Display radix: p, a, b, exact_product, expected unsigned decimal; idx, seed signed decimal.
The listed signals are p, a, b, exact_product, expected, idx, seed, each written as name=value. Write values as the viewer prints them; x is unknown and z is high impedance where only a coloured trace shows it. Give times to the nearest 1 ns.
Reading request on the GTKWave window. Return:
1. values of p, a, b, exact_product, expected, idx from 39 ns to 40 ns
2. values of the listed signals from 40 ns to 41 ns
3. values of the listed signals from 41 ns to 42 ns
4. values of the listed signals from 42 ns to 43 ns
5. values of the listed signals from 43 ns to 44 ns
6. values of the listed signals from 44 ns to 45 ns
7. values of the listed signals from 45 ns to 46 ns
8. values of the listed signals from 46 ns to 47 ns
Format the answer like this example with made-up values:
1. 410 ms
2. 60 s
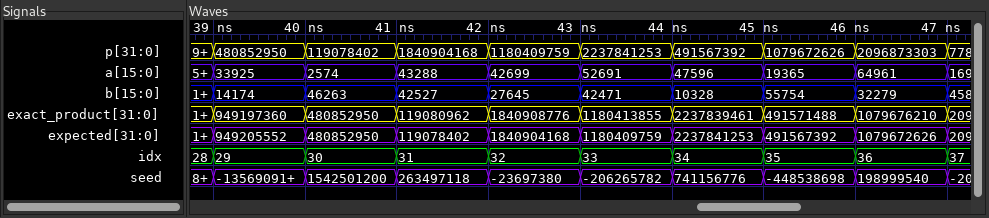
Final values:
1. p=480852950, a=33925, b=14174, exact_product=949197360, expected=949205552, idx=29
2. p=119078402, a=2574, b=46263, exact_product=480852950, expected=480852950, idx=30, seed=1542501200
3. p=1840904168, a=43288, b=42527, exact_product=119080962, expected=119078402, idx=31, seed=263497118
4. p=1180409759, a=42699, b=27645, exact_product=1840908776, expected=1840904168, idx=32, seed=-23697380
5. p=2237841253, a=52691, b=42471, exact_product=1180413855, expected=1180409759, idx=33, seed=-206265782
6. p=491567392, a=47596, b=10328, exact_product=2237839461, expected=2237841253, idx=34, seed=741156776
7. p=1079672626, a=19365, b=55754, exact_product=491571488, expected=491567392, idx=35, seed=-448538698
8. p=2096873303, a=64961, b=32279, exact_product=1079676210, expected=1079672626, idx=36, seed=198999540
